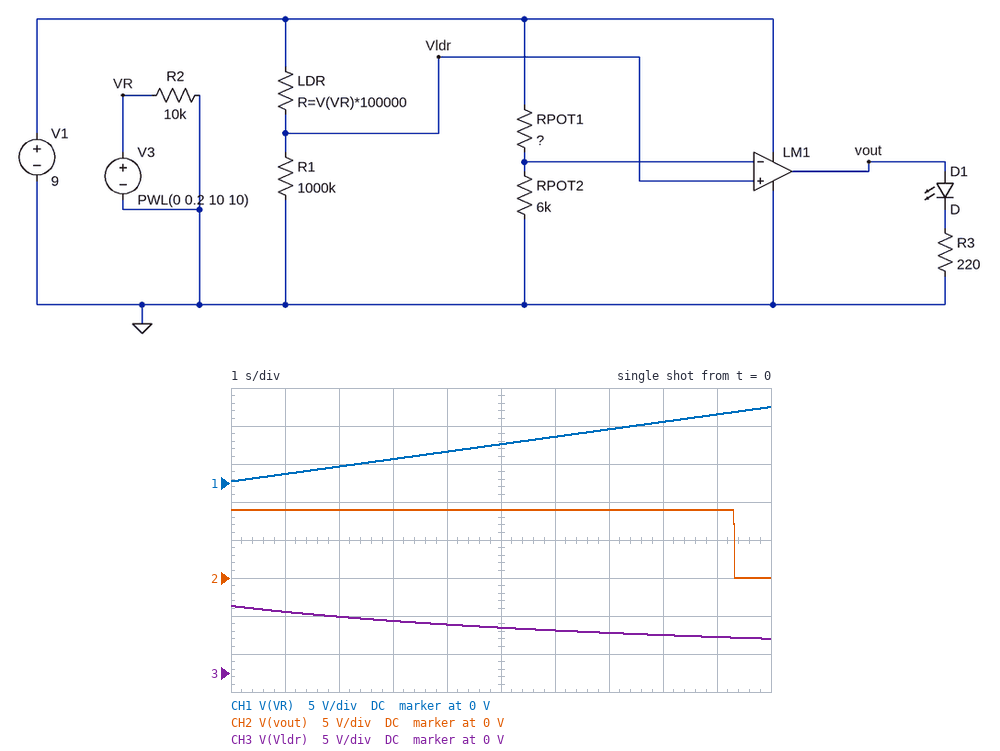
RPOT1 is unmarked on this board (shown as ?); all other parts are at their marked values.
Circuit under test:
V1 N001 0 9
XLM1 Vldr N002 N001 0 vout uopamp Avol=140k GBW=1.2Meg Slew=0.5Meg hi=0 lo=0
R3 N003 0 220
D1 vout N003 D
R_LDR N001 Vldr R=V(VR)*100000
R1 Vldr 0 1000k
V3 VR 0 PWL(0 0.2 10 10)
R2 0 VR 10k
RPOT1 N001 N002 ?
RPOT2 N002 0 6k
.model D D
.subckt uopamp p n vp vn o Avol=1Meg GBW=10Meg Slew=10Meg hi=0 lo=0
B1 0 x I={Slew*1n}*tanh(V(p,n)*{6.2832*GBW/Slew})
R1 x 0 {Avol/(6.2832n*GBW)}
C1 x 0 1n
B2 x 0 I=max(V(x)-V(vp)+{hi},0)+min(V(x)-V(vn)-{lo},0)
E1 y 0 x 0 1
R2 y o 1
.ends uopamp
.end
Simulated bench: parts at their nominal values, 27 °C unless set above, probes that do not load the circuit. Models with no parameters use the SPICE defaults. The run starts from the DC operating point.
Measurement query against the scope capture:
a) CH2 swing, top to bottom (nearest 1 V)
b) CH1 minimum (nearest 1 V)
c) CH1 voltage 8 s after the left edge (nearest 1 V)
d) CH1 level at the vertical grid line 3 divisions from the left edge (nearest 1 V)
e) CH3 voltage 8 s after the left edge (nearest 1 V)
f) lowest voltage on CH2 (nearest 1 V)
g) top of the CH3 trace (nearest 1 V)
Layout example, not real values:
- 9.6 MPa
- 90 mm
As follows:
- 9 V
- 0 V
- 8 V
- 3 V
- 5 V
- 0 V
- 9 V
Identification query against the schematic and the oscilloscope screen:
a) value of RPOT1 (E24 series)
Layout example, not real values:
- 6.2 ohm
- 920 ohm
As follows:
- 5.6 kΩ
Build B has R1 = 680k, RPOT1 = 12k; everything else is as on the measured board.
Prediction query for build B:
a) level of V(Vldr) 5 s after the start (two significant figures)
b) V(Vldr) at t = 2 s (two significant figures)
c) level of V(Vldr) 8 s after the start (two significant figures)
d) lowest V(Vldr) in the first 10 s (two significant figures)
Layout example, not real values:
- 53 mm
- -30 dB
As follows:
- 5.1 V
- 6.8 V
- 4.1 V
- 3.6 V
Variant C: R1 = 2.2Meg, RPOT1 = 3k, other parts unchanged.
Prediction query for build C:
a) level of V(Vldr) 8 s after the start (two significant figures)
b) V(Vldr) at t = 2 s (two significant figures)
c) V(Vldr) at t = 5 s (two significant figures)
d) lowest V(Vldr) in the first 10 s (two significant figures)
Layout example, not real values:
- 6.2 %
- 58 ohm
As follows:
- 6.6 V
- 8.2 V
- 7.3 V
- 6.2 V
